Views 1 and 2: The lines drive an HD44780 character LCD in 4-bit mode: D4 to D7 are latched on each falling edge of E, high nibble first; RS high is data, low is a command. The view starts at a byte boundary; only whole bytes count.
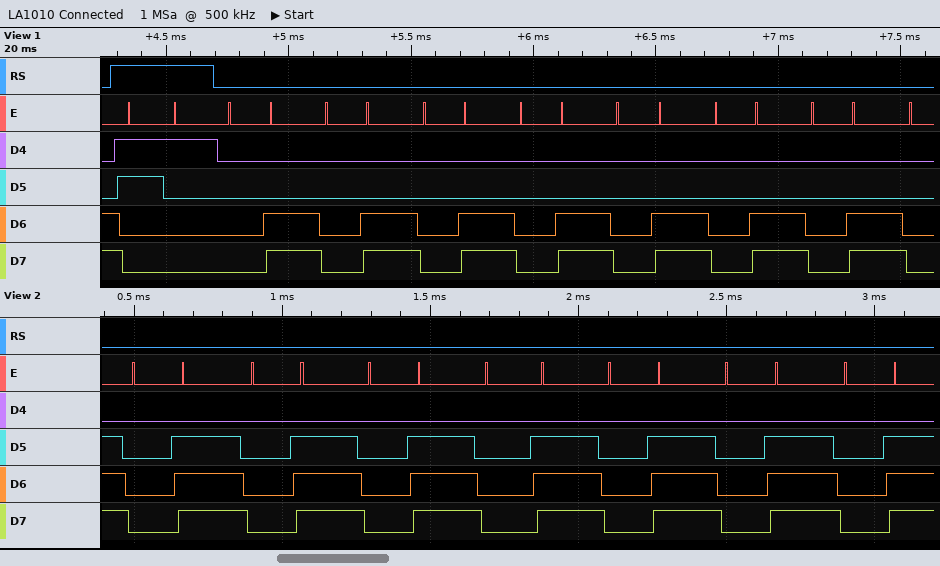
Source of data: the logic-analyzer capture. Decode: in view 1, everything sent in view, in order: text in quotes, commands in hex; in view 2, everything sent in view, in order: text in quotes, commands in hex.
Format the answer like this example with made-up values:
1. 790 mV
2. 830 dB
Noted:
1. "1" 0x0C 0x0C 0x0C 0x0C 0x0C 0x0C 0x0C
2. 0x0E 0x0E 0x0E 0x0E 0x0E 0x0E 0x0E
